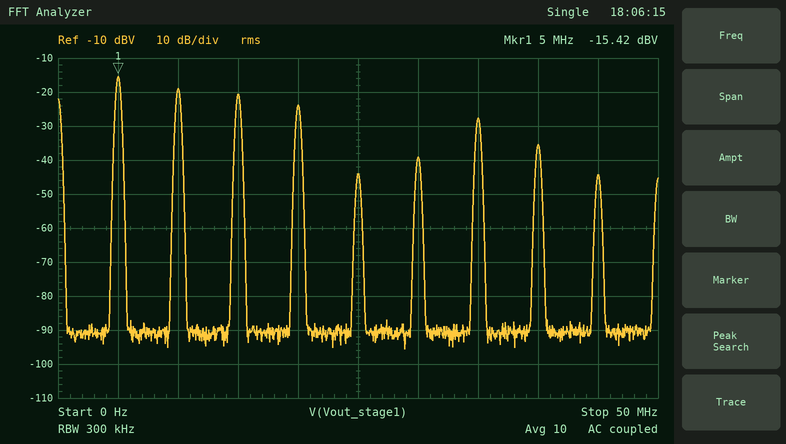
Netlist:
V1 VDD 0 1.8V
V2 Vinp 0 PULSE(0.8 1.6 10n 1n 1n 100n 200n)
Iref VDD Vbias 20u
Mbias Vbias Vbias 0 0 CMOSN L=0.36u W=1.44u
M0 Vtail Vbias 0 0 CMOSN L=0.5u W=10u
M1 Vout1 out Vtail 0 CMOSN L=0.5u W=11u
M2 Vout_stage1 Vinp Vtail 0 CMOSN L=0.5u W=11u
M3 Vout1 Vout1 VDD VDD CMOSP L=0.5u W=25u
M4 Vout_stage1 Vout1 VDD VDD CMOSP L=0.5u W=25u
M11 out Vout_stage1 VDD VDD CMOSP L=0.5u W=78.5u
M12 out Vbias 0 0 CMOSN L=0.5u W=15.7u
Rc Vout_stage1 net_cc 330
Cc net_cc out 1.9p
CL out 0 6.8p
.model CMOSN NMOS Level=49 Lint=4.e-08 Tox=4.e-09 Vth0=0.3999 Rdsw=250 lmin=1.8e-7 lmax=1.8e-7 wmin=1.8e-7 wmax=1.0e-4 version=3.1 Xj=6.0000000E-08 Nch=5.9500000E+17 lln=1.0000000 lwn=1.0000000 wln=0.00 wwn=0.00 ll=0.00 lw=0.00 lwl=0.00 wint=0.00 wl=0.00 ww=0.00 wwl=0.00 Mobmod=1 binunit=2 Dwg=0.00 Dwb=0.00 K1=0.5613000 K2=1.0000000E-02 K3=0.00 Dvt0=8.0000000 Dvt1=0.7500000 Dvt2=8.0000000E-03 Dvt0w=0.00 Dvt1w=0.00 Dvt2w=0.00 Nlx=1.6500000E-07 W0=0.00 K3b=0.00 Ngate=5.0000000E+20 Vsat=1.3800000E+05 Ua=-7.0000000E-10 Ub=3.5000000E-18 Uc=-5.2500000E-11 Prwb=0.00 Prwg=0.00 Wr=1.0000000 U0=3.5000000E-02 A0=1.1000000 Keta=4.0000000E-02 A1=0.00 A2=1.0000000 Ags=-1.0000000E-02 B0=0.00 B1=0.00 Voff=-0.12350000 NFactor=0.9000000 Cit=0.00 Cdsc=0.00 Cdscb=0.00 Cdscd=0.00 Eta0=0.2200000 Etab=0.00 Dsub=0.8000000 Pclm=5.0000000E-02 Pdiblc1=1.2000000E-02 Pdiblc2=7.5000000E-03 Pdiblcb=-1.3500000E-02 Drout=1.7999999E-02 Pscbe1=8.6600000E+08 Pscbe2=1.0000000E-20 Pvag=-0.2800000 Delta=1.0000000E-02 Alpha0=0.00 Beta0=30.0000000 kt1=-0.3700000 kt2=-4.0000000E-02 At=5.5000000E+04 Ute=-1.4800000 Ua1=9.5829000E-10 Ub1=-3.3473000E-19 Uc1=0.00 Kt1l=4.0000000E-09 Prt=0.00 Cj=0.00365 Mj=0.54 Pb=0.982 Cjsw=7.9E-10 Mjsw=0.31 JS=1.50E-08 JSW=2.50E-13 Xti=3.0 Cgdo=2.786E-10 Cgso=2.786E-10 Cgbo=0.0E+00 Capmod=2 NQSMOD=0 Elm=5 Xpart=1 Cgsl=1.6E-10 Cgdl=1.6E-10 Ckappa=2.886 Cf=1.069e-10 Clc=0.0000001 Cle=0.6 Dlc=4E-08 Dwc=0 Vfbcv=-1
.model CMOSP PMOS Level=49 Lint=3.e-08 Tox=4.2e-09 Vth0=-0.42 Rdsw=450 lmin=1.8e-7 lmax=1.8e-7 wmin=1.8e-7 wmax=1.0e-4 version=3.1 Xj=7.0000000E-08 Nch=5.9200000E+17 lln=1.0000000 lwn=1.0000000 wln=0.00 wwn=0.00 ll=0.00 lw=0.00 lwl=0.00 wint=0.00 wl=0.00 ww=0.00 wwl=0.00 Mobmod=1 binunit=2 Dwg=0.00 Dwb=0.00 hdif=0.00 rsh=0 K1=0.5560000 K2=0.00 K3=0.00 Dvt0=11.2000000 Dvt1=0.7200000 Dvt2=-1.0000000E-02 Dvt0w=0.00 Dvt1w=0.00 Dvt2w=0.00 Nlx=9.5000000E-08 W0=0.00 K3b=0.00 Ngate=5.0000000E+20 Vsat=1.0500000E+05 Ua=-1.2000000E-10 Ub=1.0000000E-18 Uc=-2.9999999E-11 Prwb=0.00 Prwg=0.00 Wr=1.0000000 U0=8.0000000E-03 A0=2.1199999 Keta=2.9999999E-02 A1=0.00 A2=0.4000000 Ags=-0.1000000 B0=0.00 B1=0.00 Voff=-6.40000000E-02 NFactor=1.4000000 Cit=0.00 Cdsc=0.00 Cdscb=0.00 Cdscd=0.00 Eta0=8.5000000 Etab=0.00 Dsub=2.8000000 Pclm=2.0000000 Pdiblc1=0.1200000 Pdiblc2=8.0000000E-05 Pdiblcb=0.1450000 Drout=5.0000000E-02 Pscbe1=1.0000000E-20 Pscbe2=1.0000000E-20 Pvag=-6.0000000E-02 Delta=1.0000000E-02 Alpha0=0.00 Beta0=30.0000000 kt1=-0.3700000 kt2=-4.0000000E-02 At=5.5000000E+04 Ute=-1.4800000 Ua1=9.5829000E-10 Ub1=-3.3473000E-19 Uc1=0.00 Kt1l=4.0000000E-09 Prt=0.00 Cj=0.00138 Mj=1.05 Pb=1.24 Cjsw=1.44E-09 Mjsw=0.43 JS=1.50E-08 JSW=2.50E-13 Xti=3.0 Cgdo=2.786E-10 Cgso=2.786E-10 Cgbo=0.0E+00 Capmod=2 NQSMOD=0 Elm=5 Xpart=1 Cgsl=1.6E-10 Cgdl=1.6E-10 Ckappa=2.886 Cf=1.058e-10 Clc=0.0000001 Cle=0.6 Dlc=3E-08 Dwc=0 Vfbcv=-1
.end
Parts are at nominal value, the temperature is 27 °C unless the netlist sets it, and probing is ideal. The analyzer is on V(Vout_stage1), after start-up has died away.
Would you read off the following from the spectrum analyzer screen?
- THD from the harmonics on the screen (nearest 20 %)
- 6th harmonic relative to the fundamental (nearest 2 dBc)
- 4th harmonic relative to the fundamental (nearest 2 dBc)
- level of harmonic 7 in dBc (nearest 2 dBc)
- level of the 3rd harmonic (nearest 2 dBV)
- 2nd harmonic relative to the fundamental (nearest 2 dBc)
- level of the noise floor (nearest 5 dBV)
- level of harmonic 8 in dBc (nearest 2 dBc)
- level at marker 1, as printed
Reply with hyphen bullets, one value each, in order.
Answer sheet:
- 100 %
- -24 dBc
- -8 dBc
- -12 dBc
- -20 dBV
- -4 dBc
- -90 dBV
- -20 dBc
- -15.42 dBV
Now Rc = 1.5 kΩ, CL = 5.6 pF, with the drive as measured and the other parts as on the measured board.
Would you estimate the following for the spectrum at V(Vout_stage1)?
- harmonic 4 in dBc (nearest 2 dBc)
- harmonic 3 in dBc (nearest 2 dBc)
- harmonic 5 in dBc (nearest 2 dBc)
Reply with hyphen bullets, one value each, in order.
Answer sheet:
- -6 dBc
- -4 dBc
- -16 dBc
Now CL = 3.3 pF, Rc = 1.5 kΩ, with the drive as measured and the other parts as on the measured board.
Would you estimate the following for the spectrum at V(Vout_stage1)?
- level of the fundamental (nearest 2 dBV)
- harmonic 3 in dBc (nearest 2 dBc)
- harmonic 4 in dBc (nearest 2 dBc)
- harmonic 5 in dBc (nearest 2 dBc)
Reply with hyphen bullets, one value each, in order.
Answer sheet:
- -22 dBV
- -2 dBc
- -6 dBc
- -6 dBc
